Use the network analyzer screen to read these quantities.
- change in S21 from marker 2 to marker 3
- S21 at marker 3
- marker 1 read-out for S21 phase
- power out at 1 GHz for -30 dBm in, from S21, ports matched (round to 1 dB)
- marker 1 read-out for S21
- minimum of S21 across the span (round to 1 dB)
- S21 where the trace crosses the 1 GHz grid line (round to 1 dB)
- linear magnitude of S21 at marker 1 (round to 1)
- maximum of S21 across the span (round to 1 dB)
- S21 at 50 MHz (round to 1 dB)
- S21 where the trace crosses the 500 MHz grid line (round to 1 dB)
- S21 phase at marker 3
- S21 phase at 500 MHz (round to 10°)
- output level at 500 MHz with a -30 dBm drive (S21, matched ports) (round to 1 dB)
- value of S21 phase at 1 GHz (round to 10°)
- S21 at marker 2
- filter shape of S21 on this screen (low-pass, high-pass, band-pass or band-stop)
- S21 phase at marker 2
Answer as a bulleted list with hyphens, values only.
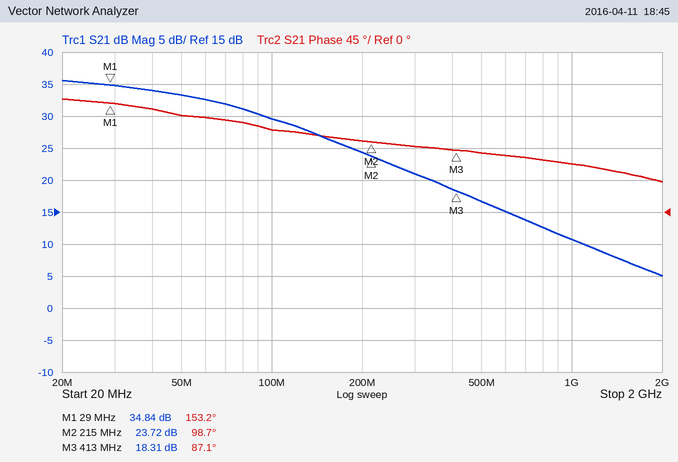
- -5.41 dB
- 18.31 dB
- 153.2°
- -19 dBm
- 34.84 dB
- 5 dB
- 11 dB
- 55
- 36 dB
- 33 dB
- 17 dB
- 87.1°
- 80°
- -13 dBm
- 70°
- 23.72 dB
- low-pass
- 98.7°
